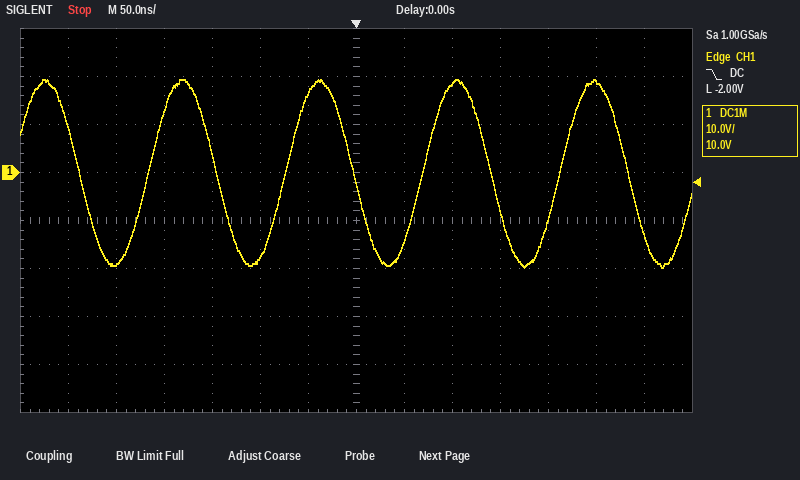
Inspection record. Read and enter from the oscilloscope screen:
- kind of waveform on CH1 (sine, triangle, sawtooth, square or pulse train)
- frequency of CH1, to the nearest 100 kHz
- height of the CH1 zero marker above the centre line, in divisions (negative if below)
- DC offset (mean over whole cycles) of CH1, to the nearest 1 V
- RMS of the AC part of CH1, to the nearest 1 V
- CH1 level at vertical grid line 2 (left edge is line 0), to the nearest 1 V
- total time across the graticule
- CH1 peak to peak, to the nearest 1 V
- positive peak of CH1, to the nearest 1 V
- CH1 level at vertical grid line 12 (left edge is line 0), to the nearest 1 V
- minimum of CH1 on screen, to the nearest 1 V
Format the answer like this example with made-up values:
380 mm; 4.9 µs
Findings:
sine; 7.0 MHz; +1.0 div; 0 V; 14 V; -19 V; 700 ns; 39 V; 19 V; 19 V; -20 V
